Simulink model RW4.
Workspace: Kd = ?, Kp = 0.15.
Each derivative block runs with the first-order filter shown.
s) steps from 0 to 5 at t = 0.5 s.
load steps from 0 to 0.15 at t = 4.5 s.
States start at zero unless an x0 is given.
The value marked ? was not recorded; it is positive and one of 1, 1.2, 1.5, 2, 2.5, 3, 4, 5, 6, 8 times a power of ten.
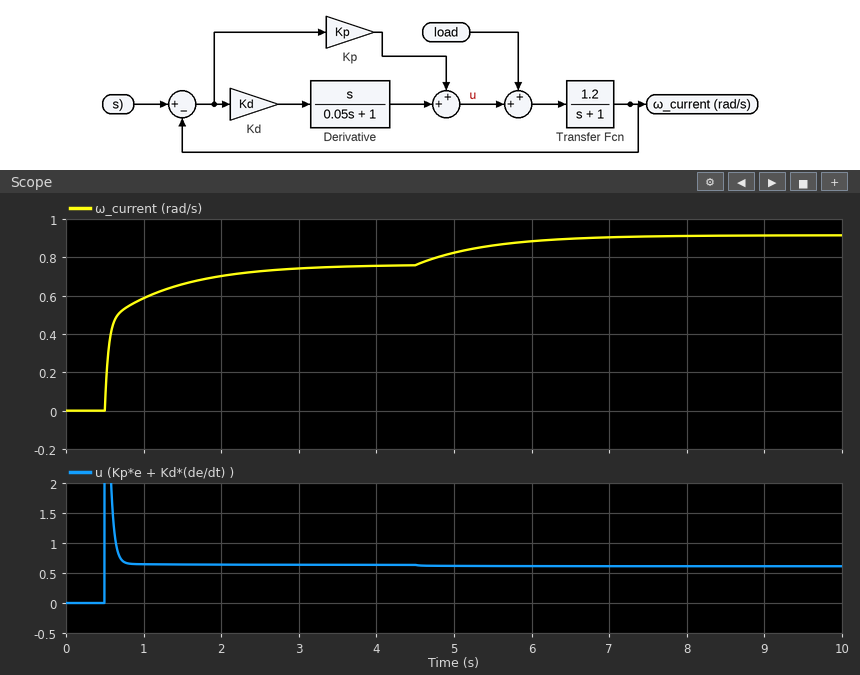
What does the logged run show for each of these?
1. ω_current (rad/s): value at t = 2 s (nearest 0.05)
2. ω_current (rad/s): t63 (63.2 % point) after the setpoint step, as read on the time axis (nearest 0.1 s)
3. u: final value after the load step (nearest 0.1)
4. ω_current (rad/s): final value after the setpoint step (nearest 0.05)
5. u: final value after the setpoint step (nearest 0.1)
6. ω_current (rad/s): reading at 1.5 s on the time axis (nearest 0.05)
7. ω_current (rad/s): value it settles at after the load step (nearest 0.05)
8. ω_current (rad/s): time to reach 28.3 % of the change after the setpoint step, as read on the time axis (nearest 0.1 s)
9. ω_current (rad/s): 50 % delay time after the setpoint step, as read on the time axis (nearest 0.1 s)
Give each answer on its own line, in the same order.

0.70
0.6 s
0.6
0.75
0.6
0.65
0.90
0.5 s
0.6 s
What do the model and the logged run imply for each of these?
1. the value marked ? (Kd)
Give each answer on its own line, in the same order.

0.08
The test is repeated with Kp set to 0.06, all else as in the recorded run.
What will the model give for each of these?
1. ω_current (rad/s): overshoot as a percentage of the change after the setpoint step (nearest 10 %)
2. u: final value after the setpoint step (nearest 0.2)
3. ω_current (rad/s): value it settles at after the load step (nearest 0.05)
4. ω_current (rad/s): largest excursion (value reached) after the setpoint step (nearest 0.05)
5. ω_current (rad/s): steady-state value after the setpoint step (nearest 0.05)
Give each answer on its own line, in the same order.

30 %
0.2
0.50
0.45
0.35
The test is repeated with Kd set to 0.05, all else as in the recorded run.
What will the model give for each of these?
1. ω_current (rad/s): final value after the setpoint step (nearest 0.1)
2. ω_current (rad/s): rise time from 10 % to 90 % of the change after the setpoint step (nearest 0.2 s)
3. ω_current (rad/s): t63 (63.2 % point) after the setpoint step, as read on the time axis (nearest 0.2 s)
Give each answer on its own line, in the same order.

0.8
1.6 s
1.0 s
